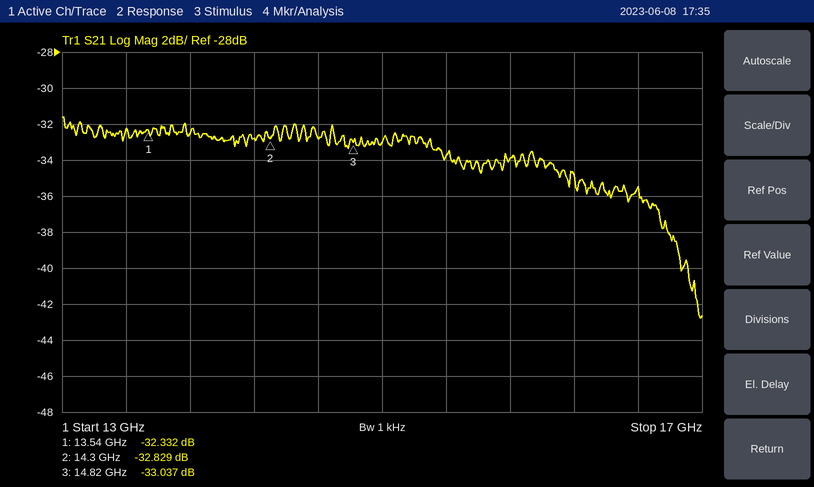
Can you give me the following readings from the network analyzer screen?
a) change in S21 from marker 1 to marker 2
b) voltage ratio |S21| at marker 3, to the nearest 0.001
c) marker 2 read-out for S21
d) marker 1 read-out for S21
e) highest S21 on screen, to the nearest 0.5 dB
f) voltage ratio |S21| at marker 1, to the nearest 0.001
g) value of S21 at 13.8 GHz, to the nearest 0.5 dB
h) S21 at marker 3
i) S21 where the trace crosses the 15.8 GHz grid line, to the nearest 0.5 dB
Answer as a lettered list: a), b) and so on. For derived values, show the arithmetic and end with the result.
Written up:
a) -32.829 − (-32.332) = -0.497 dB
b) 10^(-33.037/20) ≈ 0.022
c) -32.829 dB
d) -32.332 dB
e) -31.5 dB
f) 10^(-32.332/20) ≈ 0.024
g) -32.5 dB
h) -33.037 dB
i) -34.0 dB
